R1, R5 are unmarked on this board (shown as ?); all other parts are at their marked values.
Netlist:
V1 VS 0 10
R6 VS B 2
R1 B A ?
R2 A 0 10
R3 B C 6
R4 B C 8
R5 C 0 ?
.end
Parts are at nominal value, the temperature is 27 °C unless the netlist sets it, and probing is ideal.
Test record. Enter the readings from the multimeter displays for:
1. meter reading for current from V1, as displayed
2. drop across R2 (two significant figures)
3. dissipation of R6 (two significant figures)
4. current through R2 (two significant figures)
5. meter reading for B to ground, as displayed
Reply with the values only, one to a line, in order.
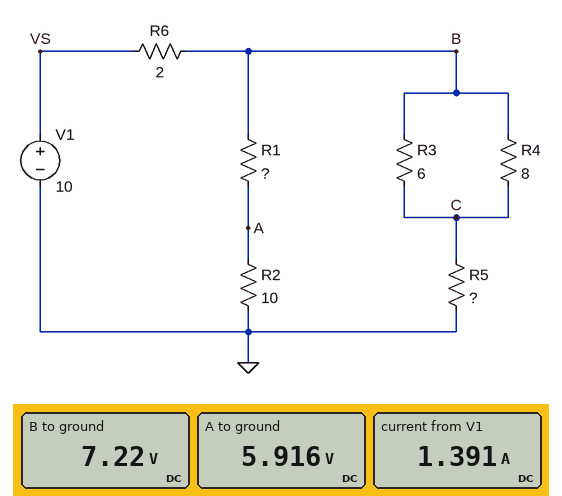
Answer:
1.391 A
5.9 V
3.9 W
590 mA
7.22 V
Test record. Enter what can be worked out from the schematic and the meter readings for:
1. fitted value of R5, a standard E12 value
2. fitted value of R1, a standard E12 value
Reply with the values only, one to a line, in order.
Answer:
5.6 Ω
2.2 Ω
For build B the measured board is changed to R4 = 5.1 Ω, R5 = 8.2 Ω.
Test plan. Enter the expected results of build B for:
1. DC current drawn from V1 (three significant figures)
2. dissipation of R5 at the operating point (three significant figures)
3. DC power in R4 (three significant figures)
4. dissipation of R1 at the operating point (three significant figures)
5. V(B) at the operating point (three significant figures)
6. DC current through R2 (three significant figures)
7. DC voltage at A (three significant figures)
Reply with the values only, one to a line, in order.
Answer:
1.29 A
3.77 W
685 mW
815 mW
7.43 V
609 mA
6.09 V
